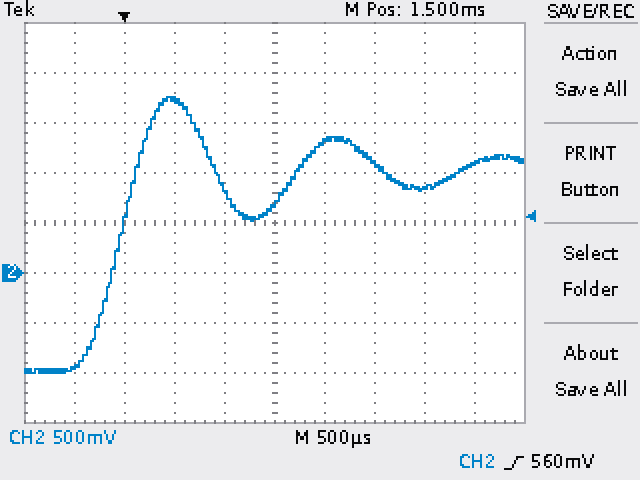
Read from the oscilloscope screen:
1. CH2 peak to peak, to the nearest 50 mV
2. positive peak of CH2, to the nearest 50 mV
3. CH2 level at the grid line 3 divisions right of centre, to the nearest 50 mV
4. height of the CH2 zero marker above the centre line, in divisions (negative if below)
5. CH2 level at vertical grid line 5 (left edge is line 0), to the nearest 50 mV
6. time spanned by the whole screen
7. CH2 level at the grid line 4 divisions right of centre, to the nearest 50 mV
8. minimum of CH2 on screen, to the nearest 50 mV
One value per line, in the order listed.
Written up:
2.75 V
1.75 V
850 mV
-1.0 div
650 mV
5 ms
1.10 V
-1.00 V
